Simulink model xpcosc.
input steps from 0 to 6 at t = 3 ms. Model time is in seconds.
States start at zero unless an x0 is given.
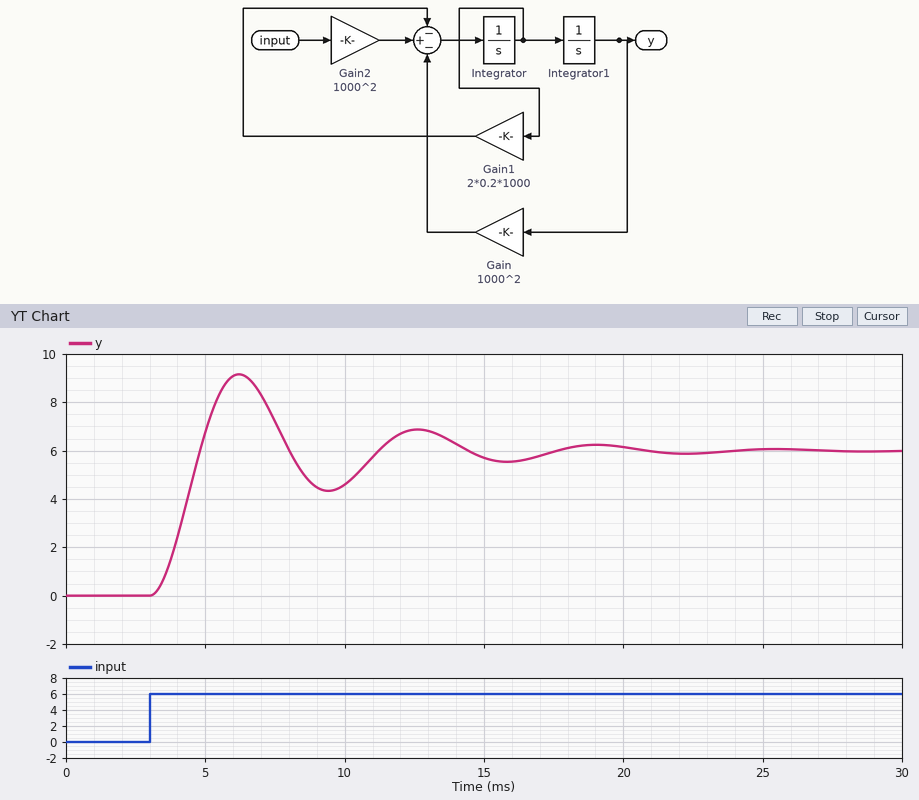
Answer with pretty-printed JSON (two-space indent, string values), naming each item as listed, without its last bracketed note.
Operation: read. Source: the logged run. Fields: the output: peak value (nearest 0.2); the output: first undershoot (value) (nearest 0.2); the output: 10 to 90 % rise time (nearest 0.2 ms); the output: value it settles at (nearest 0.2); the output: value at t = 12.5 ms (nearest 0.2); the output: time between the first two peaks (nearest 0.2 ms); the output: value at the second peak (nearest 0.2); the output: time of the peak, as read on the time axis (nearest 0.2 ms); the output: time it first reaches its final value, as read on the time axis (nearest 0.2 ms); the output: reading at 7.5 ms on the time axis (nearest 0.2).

{
  "the output: peak value": "9.2",
  "the output: first undershoot (value)": "4.4",
  "the output: 10 to 90 % rise time": "1.2 ms",
  "the output: value it settles at": "6.0",
  "the output: value at t = 12.5 ms": "6.8",
  "the output: time between the first two peaks": "6.4 ms",
  "the output: value at the second peak": "6.8",
  "the output: time of the peak, as read on the time axis": "6.2 ms",
  "the output: time it first reaches its final value, as read on the time axis": "4.8 ms",
  "the output: reading at 7.5 ms on the time axis": "7.2"
}
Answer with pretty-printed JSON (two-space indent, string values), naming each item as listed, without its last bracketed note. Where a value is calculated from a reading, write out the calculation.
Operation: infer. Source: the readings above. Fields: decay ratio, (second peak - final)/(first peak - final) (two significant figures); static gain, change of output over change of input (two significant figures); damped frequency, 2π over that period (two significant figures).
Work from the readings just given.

{
  "decay ratio, (second peak - final)/(first peak - final)": "(6.8 - 6) / (9.2 - 6) = 0.25",
  "static gain, change of output over change of input": "(6 - 0) / (6 - 0) = 1.0",
  "damped frequency, 2π over that period": "2π / 6.4 = 0.98 rad/ms"
}
